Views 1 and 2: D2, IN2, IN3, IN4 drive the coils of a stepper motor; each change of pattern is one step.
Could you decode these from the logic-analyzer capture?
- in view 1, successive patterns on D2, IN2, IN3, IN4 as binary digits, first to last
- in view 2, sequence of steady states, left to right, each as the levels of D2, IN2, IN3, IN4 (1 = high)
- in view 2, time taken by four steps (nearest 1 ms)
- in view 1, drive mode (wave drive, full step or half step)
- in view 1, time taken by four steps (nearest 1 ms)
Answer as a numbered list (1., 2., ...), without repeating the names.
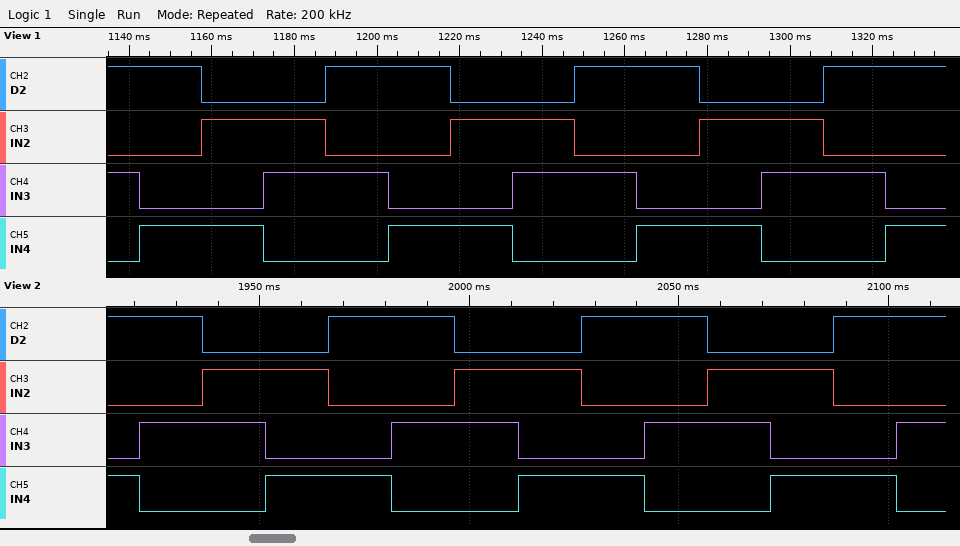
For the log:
1. 1010 1001 0101 0110 1010 1001 0101 0110 1010 1001 0101 0110 1010 1001
2. 1001 1010 0110 0101 1001 1010 0110 0101 1001 1010 0110 0101 1001 1010
3. 60 ms
4. full step
5. 60 ms
